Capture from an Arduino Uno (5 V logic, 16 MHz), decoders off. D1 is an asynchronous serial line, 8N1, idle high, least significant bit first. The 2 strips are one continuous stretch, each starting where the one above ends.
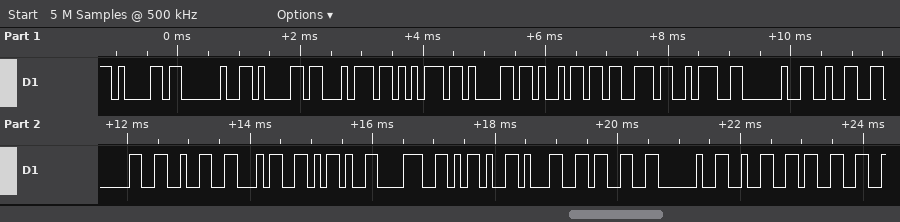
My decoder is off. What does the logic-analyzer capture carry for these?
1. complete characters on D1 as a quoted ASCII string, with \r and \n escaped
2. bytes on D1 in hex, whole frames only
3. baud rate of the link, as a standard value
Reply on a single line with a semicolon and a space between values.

"a atuais: 2024-8-13 23"; 61 20 61 74 75 61 69 73 3A 20 32 30 32 34 2D 38 2D 31 33 20 32 33; 9600 baud
